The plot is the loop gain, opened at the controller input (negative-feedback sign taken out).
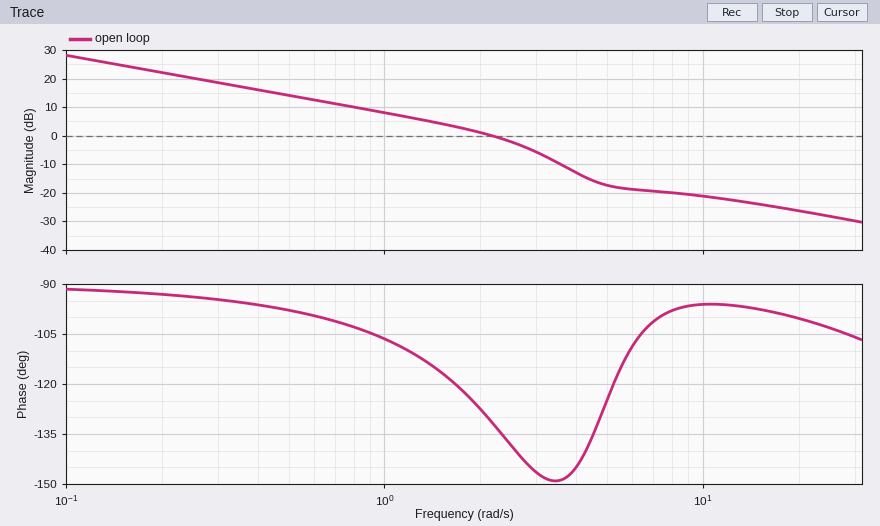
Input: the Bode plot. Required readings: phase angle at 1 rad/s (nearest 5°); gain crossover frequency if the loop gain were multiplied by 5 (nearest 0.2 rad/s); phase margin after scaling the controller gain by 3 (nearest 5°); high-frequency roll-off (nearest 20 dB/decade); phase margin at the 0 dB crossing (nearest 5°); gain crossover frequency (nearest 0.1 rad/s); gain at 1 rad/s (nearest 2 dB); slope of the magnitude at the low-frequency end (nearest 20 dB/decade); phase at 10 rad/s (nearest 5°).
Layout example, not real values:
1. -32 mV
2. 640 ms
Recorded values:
1. -105°
2. 4.2 rad/s
3. 30°
4. -20 dB/decade
5. 50°
6. 2.2 rad/s
7. 8 dB
8. -20 dB/decade
9. -95°
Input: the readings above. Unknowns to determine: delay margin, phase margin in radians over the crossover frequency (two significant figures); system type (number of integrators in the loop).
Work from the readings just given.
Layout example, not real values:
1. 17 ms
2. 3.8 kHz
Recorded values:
1. 0.40 s
2. 1
